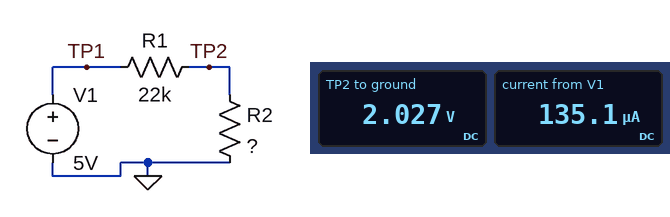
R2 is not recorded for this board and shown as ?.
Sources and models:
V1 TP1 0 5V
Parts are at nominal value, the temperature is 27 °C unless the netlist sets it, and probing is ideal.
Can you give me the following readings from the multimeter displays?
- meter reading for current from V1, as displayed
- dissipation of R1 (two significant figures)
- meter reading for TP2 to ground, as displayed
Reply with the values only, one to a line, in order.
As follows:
135.1 µA
400 µW
2.027 V
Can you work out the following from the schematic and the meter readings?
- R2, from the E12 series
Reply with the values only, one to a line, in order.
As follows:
15 kΩ
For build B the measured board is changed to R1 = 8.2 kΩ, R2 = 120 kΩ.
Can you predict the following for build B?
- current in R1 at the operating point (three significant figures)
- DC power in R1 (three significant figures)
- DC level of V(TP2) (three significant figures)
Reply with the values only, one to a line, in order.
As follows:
39.0 µA
12.5 µW
4.68 V
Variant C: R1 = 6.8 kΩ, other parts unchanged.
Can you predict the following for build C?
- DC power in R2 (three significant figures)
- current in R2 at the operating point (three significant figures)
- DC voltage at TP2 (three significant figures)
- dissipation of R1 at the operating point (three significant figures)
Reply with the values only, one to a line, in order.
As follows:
789 µW
229 µA
3.44 V
358 µW
